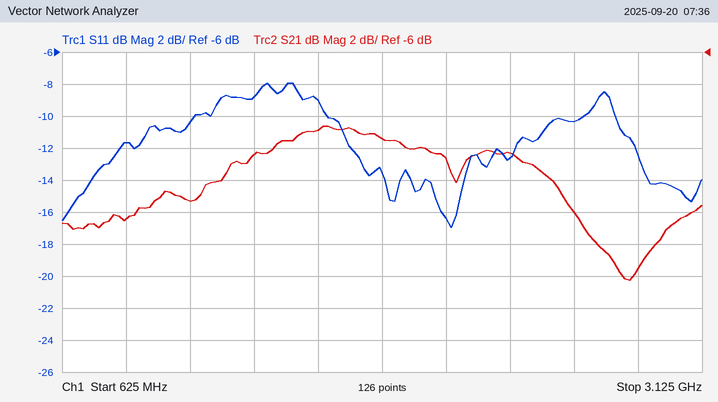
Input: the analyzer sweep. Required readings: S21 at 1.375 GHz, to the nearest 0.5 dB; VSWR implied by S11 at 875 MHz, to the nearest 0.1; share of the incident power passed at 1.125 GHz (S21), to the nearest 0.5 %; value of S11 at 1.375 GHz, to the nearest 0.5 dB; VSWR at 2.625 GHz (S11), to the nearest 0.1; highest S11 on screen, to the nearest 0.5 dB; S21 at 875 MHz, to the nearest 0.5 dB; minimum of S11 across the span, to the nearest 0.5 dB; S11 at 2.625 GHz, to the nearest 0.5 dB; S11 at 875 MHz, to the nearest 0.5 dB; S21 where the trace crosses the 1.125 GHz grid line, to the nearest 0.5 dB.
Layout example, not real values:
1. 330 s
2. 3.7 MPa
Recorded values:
1. -12.5 dB
2. 1.7
3. 3.0 %
4. -9.0 dB
5. 1.9
6. -8.0 dB
7. -16.5 dB
8. -17.0 dB
9. -10.5 dB
10. -11.5 dB
11. -15.5 dB
